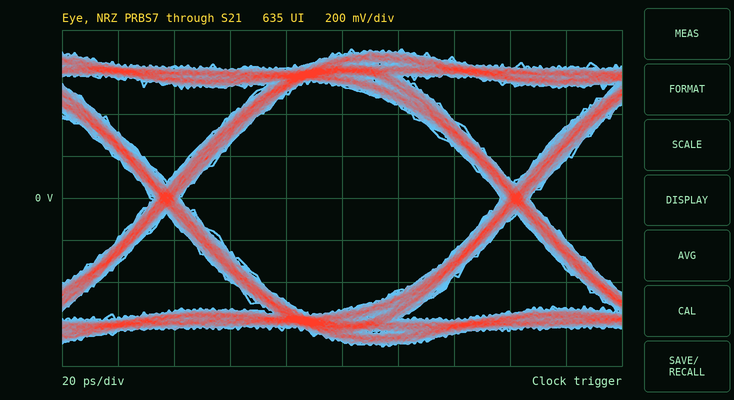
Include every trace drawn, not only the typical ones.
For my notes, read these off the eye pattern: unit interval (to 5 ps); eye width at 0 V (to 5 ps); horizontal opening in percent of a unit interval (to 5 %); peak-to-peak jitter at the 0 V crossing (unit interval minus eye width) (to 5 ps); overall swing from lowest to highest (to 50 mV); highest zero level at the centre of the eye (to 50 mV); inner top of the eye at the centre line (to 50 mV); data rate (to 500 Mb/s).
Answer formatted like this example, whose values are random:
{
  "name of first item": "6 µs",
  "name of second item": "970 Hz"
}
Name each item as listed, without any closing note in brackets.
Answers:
{
  "unit interval": "125 ps",
  "eye width at 0 V": "115 ps",
  "horizontal opening in percent of a unit interval": "90 %",
  "peak-to-peak jitter at the 0 V crossing (unit interval minus eye width)": "10 ps",
  "overall swing from lowest to highest": "1.40 V",
  "highest zero level at the centre of the eye": "-550 mV",
  "inner top of the eye at the centre line": "550 mV",
  "data rate": "8.0 Gb/s"
}
